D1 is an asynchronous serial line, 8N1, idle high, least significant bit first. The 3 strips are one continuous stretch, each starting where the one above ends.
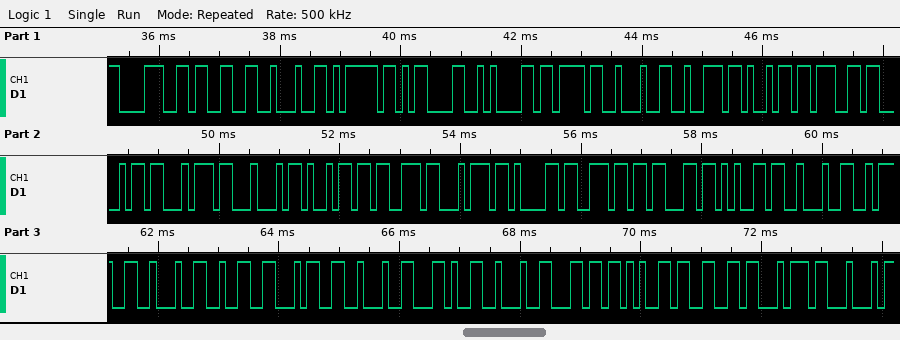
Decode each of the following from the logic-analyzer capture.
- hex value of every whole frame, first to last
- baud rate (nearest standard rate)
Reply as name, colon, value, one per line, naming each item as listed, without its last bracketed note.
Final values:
hex value of every whole frame, first to last: 38 33 22 7D 0D 0A 7B 22 72 69 67 68 74 44 69 73 74 61 6E 63 65 22 3A 22 32 34 22 2C 22 6C 65 66 74 44
baud rate: 9600 baud
